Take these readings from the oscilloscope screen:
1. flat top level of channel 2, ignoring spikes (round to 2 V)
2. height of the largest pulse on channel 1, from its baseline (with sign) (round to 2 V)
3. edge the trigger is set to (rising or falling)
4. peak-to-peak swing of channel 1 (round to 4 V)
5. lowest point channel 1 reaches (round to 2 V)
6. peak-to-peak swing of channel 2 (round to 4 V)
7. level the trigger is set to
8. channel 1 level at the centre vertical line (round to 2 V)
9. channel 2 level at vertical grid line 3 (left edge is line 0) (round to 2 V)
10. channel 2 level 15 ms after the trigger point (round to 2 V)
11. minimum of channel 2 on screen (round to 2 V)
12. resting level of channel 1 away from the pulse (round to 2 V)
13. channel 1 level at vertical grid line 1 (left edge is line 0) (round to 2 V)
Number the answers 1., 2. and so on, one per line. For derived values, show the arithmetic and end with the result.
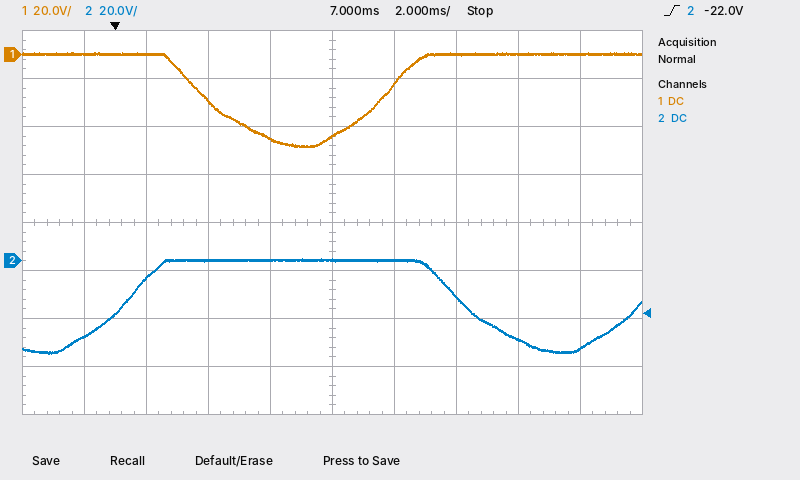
1. 0 V
2. -38 V − (0 V) = -38 V
3. rising
4. 40 V
5. -38 V
6. 40 V
7. -22.0 V
8. -34 V
9. 0 V
10. -36 V
11. -38 V
12. 0 V
13. 0 V
